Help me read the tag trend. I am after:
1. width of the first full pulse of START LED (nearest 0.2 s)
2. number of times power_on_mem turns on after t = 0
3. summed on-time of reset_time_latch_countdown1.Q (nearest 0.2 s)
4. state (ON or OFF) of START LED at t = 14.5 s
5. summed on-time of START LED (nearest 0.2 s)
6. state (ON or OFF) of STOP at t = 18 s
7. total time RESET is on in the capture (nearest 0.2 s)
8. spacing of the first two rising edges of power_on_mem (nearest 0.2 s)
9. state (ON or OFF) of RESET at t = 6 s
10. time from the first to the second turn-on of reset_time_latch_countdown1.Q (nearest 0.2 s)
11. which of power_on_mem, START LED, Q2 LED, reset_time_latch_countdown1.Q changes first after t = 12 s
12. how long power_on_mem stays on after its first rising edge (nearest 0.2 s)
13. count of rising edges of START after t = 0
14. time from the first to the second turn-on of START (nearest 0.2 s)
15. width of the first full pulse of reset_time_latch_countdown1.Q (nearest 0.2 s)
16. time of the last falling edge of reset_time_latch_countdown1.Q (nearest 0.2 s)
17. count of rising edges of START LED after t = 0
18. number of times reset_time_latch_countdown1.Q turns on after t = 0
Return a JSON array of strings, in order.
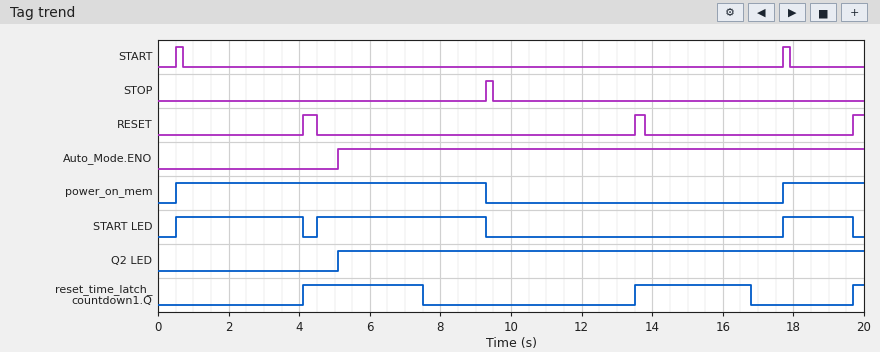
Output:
["3.6 s", "2", "7.0 s", "OFF", "10.4 s", "OFF", "1.0 s", "17.2 s", "OFF", "9.4 s", "reset_time_latch_countdown1.Q", "8.8 s", "2", "17.2 s", "3.4 s", "16.8 s", "3", "3"]
